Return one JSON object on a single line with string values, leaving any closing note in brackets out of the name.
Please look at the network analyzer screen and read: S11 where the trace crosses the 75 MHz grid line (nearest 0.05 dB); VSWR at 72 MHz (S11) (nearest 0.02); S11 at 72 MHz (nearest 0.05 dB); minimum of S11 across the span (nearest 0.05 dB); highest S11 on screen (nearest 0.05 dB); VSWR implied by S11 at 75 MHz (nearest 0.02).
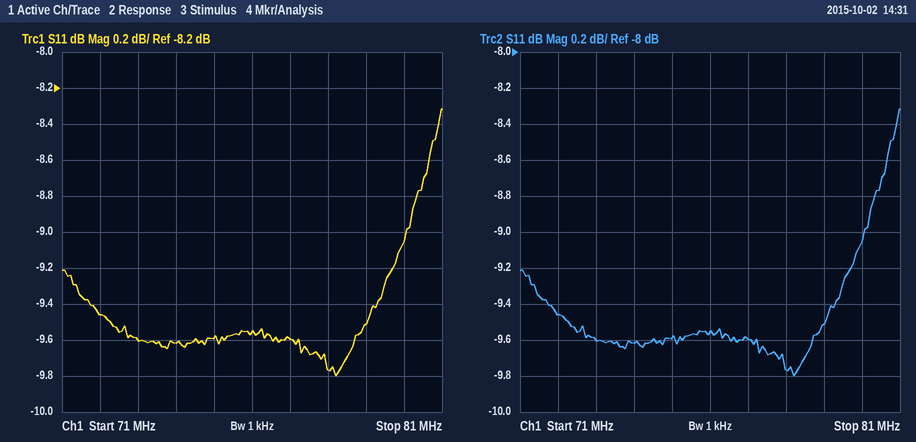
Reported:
{"S11 where the trace crosses the 75 MHz grid line": "-9.60 dB", "VSWR at 72 MHz (S11)": "2.02", "S11 at 72 MHz": "-9.45 dB", "minimum of S11 across the span": "-9.80 dB", "highest S11 on screen": "-8.30 dB", "VSWR implied by S11 at 75 MHz": "2.00"}
